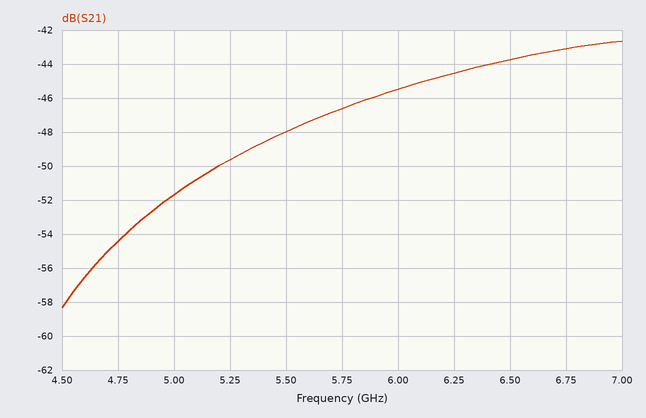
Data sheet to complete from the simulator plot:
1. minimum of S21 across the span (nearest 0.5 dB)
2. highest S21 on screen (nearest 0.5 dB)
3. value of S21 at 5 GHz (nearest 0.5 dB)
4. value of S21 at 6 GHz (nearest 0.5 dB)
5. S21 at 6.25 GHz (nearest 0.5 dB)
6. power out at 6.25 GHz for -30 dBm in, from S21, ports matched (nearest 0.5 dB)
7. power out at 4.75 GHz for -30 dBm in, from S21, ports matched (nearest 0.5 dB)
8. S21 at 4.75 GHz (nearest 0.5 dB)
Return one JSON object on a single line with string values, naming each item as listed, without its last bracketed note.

{"minimum of S21 across the span": "-58.5 dB", "highest S21 on screen": "-42.5 dB", "value of S21 at 5 GHz": "-51.5 dB", "value of S21 at 6 GHz": "-45.5 dB", "S21 at 6.25 GHz": "-44.5 dB", "power out at 6.25 GHz for -30 dBm in, from S21, ports matched": "-74.5 dBm", "power out at 4.75 GHz for -30 dBm in, from S21, ports matched": "-84.5 dBm", "S21 at 4.75 GHz": "-54.5 dB"}
